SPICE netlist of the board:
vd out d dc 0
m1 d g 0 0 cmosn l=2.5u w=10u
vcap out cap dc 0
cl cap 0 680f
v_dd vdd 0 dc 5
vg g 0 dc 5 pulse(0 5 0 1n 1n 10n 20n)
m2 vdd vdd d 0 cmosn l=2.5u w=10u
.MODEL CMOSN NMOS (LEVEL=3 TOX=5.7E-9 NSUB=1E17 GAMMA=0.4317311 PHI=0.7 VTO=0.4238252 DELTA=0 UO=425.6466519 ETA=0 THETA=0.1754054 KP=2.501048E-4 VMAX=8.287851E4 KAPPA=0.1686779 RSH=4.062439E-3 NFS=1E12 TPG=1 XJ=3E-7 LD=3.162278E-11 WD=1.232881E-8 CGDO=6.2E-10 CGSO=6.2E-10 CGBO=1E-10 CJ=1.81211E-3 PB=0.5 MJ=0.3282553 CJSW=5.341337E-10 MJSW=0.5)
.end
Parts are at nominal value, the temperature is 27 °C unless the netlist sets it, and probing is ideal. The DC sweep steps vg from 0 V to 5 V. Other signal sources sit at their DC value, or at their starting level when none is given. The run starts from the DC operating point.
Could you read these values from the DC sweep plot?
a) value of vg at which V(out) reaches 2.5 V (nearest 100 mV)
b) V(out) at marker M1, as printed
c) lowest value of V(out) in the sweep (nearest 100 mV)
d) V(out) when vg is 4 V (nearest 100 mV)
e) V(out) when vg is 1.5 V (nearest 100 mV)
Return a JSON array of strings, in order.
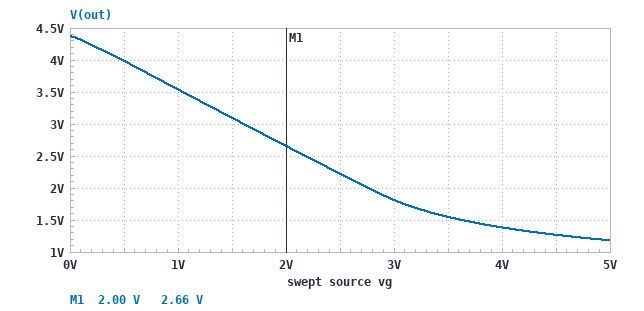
["2.2 V", "2.66 V", "1.2 V", "1.4 V", "3.1 V"]
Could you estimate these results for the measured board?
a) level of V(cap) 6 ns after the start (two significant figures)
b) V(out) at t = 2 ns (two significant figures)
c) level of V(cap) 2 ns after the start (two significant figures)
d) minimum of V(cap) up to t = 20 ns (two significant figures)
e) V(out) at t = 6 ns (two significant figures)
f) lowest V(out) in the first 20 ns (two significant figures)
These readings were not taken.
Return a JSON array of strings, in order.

["1.2 V", "1.3 V", "1.3 V", "1.2 V", "1.2 V", "1.2 V"]
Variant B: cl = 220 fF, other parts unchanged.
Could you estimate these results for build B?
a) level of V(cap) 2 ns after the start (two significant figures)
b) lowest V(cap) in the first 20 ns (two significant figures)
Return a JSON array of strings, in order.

["1.2 V", "1.1 V"]
